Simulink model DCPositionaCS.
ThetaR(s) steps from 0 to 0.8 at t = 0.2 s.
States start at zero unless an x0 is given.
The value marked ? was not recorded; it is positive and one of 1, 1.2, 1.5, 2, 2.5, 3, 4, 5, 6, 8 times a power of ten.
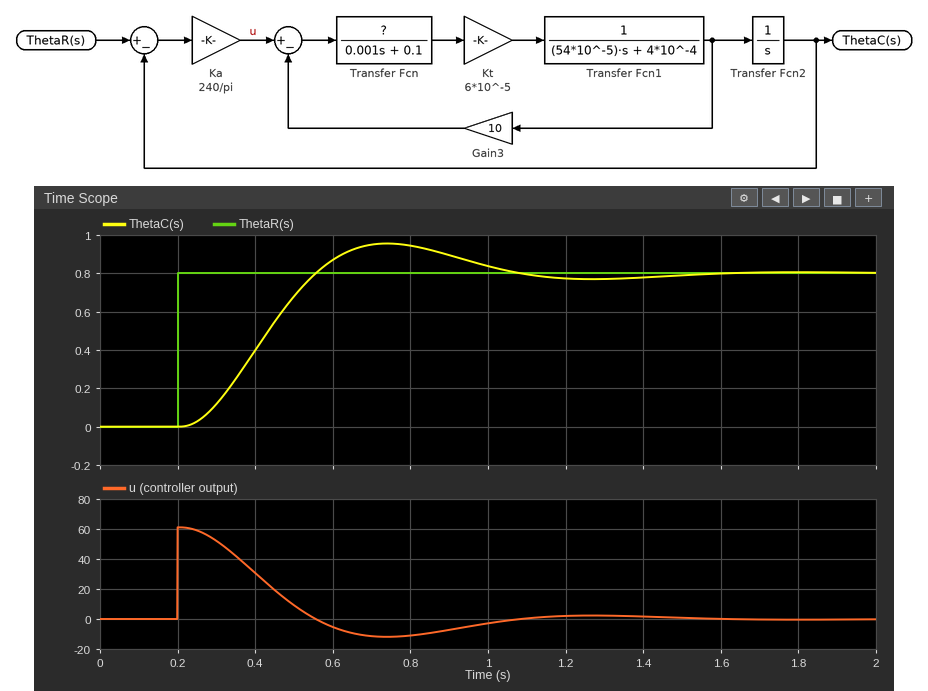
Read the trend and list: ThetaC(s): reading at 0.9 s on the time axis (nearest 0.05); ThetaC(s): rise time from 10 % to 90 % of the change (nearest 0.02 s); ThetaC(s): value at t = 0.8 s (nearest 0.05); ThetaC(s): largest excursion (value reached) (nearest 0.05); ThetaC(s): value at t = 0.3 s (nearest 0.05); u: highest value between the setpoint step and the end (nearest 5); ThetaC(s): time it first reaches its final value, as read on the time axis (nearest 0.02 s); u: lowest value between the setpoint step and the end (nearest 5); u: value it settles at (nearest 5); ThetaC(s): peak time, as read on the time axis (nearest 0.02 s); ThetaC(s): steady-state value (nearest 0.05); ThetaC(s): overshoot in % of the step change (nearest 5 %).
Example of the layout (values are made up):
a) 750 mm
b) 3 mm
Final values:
a) 0.90
b) 0.24 s
c) 0.95
d) 0.95
e) 0.10
f) 60
g) 0.56 s
h) -10
i) 0
j) 0.74 s
k) 0.80
l) 20 %
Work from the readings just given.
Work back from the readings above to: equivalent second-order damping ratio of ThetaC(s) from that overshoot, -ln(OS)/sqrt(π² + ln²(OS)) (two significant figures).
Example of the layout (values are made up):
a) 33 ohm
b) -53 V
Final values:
a) 0.46
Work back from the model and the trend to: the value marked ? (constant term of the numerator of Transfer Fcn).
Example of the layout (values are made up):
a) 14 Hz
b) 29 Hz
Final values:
a) 0.5
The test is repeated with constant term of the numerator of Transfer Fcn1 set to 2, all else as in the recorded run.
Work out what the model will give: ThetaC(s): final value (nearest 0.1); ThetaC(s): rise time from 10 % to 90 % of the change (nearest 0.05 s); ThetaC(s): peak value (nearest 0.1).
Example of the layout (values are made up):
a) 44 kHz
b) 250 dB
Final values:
a) 0.8
b) 0.20 s
c) 0.9
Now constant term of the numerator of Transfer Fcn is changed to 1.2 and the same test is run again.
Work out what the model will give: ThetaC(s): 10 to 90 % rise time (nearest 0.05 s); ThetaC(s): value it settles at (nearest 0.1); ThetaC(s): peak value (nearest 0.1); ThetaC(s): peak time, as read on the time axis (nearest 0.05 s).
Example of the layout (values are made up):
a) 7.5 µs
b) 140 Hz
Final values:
a) 0.20 s
b) 0.8
c) 0.8
d) 0.60 s
